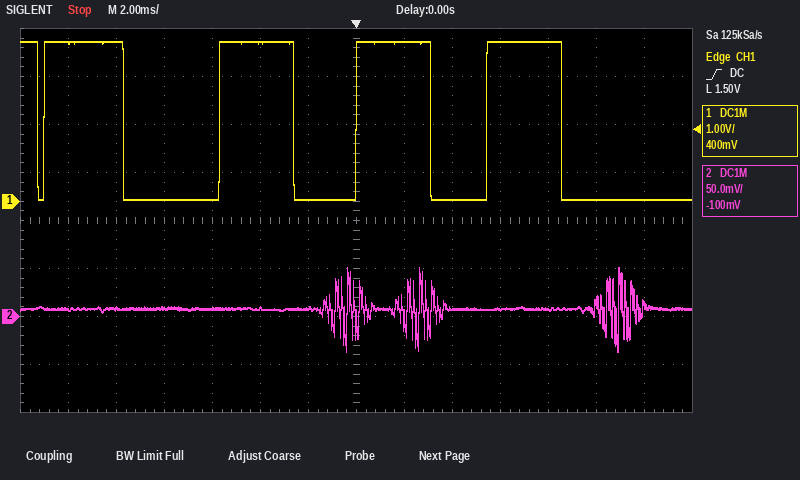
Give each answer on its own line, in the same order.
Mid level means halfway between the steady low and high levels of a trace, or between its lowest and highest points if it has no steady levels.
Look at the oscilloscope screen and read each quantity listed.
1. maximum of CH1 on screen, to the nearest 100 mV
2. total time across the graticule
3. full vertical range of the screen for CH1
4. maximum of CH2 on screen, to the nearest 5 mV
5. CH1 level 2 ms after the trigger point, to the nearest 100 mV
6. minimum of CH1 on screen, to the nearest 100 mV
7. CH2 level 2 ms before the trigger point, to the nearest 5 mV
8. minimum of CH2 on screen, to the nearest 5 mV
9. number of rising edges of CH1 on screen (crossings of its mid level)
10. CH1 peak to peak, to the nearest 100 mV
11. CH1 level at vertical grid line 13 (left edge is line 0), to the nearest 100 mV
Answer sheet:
3.3 V
28 ms
8 V
50 mV
3.3 V
0.0 V
10 mV
-35 mV
4
3.3 V
0.0 V
